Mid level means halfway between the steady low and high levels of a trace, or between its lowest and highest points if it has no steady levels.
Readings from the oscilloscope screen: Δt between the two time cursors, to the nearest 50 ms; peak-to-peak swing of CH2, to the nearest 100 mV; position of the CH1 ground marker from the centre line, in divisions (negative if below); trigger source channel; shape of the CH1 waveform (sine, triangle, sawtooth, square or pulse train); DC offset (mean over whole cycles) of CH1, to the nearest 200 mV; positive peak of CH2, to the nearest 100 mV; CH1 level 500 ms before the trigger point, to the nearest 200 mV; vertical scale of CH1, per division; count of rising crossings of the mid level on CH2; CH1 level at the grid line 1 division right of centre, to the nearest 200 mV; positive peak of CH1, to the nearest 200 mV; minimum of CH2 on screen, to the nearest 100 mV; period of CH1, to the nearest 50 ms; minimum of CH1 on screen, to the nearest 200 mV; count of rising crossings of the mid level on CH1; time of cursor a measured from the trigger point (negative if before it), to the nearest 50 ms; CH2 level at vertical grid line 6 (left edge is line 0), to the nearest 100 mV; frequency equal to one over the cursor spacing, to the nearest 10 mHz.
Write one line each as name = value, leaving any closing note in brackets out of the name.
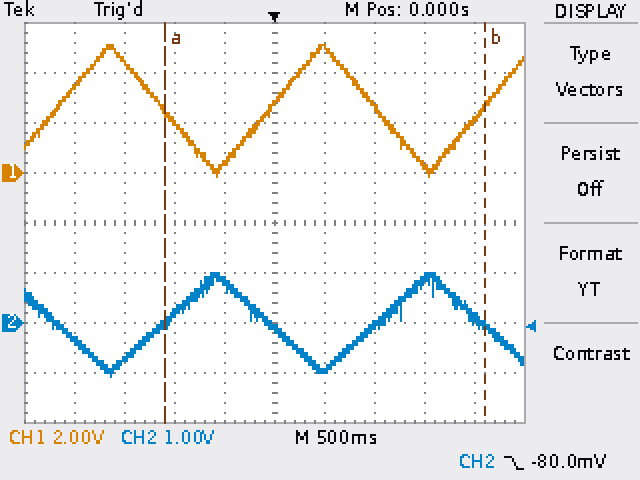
Δt between the two time cursors, to the nearest 50 ms = 3.20 s
peak-to-peak swing of CH2, to the nearest 100 mV = 2.1 V
position of the CH1 ground marker from the centre line, in divisions = +1.0 div
trigger source channel = CH2
shape of the CH1 waveform = triangle
DC offset (mean over whole cycles) of CH1, to the nearest 200 mV = 2.6 V
positive peak of CH2, to the nearest 100 mV = 1.0 V
CH1 level 500 ms before the trigger point, to the nearest 200 mV = 400 mV
vertical scale of CH1, per division = 2 V
count of rising crossings of the mid level on CH2 = 2
CH1 level at the grid line 1 division right of centre, to the nearest 200 mV = 5.0 V
positive peak of CH1, to the nearest 200 mV = 5.2 V
minimum of CH2 on screen, to the nearest 100 mV = -1.1 V
period of CH1, to the nearest 50 ms = 2.15 s
minimum of CH1 on screen, to the nearest 200 mV = -200 mV
count of rising crossings of the mid level on CH1 = 3
time of cursor a measured from the trigger point (negative if before it), to the nearest 50 ms = -1.10 s
CH2 level at vertical grid line 6 (left edge is line 0), to the nearest 100 mV = -900 mV
frequency equal to one over the cursor spacing, to the nearest 10 mHz = 310 mHz
